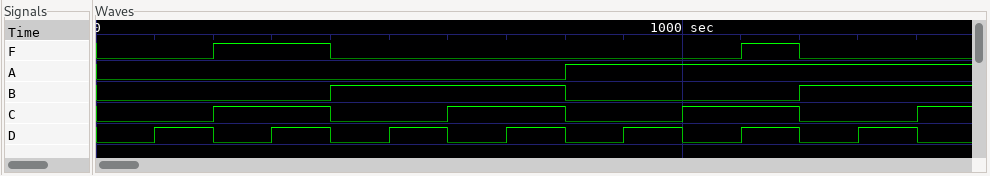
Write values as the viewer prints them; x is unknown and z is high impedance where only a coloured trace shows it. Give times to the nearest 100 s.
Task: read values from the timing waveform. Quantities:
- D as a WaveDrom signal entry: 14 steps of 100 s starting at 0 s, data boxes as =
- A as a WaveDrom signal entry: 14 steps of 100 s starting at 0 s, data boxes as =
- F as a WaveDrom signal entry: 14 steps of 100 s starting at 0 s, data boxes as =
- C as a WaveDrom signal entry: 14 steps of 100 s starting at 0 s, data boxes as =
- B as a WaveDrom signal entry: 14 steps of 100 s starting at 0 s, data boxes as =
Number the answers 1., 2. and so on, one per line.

1. {name: 'D', wave: '01010101010101'}
2. {name: 'A', wave: '0.......1.....'}
3. {name: 'F', wave: '0.1.0......10.'}
4. {name: 'C', wave: '0.1.0.1.0.1.0.'}
5. {name: 'B', wave: '0...1...0...1.'}
